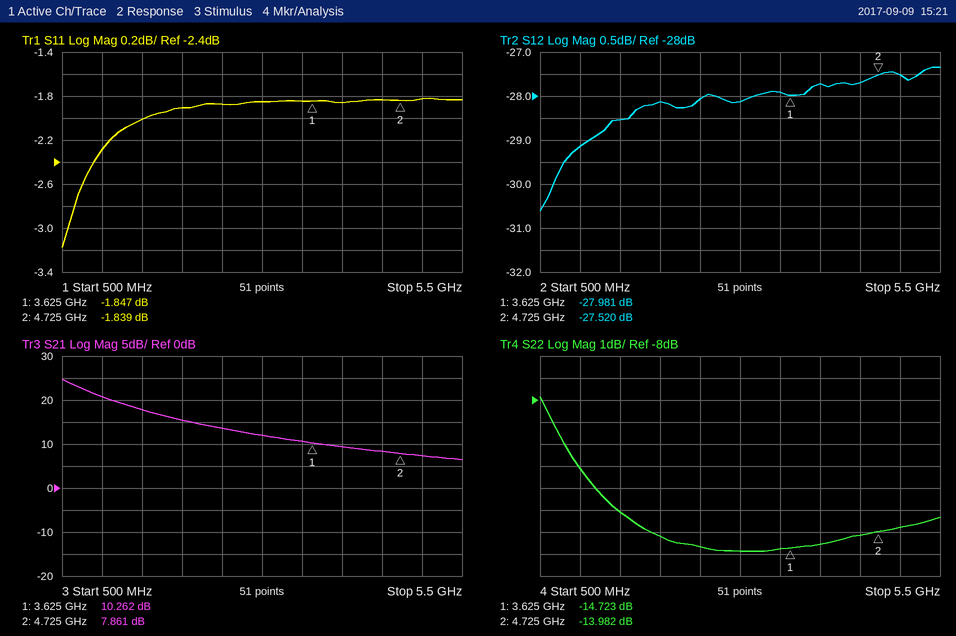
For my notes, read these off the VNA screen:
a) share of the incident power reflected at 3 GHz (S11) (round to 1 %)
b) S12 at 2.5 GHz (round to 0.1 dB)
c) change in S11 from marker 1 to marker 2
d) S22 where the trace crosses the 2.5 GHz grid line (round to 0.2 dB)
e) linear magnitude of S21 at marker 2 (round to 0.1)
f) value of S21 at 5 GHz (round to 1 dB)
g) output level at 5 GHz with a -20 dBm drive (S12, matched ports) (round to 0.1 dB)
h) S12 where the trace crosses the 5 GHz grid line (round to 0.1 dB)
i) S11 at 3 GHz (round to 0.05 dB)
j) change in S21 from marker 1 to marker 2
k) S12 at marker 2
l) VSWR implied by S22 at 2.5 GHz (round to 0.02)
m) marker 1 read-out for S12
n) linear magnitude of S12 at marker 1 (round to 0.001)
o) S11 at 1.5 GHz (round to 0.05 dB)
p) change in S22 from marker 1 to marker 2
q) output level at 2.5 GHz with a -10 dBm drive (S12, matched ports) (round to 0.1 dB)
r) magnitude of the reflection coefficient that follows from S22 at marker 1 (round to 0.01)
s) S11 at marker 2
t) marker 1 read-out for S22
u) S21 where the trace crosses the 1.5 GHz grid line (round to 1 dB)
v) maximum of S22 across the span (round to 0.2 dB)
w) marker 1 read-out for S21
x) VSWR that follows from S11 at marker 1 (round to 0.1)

65 %
-28.1 dB
0.008 dB
-14.6 dB
2.5
7 dB
-47.5 dBm
-27.5 dB
-1.85 dB
-2.401 dB
-27.520 dB
1.46
-27.981 dB
0.040
-2.00 dB
0.741 dB
-38.1 dBm
0.18
-1.839 dB
-14.723 dB
18 dB
-7.8 dB
10.262 dB
9.4
